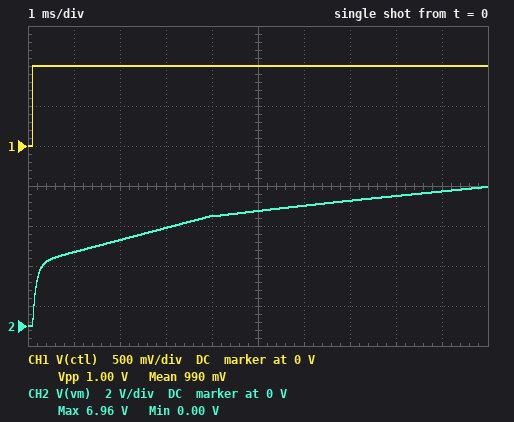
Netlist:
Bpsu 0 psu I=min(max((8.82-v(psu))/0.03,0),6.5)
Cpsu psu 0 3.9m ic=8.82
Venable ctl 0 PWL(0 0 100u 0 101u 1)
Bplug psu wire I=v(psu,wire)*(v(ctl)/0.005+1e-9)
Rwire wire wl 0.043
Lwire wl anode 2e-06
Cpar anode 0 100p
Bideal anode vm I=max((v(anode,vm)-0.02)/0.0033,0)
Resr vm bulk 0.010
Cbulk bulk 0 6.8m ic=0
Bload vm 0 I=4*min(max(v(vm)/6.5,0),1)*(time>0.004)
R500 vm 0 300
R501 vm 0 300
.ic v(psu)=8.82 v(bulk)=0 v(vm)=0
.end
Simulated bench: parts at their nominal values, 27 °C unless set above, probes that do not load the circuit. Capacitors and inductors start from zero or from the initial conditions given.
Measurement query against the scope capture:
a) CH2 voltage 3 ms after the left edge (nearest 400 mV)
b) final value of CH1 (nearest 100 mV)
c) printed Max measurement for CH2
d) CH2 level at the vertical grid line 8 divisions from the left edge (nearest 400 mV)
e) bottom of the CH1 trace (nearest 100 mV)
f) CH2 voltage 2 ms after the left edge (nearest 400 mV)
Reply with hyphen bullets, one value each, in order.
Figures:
- 4.8 V
- 1.0 V
- 6.96 V
- 6.4 V
- 0 V
- 4.4 V
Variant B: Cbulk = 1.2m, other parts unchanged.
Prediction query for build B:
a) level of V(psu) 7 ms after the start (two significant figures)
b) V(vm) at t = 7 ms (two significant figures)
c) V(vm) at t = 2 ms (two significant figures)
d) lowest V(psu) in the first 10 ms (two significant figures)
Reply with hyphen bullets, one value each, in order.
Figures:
- 8.7 V
- 8.5 V
- 8.8 V
- 6.8 V
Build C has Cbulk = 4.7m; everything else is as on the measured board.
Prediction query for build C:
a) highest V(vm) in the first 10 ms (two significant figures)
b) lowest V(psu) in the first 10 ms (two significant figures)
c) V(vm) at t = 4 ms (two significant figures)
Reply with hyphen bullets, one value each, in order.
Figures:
- 8.4 V
- 4.5 V
- 6.8 V
